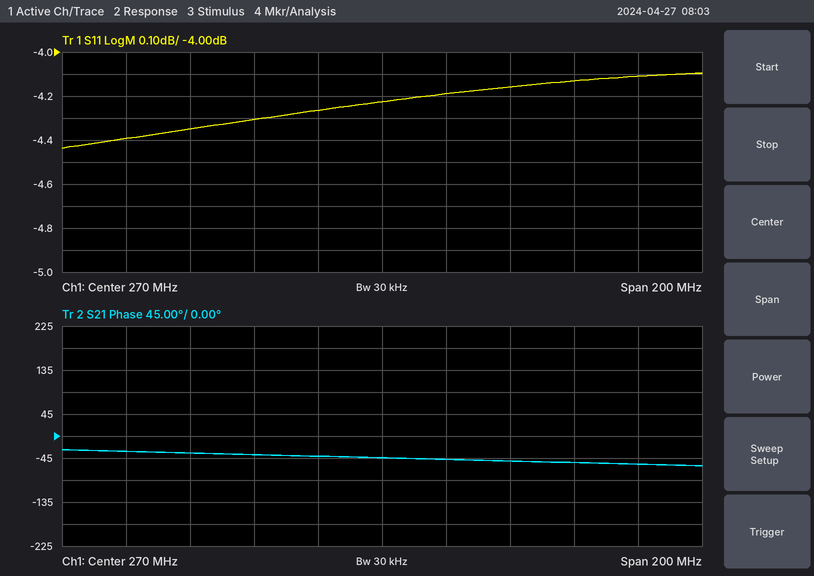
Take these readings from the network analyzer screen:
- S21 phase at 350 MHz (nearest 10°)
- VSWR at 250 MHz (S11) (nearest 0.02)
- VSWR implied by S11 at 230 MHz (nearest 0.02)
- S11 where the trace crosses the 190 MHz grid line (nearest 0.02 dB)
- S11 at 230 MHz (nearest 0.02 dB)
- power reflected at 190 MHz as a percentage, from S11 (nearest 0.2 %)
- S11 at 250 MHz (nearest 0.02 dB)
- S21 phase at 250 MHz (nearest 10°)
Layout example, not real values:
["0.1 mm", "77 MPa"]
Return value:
["-60°", "4.16", "4.12", "-4.40 dB", "-4.30 dB", "36.4 %", "-4.26 dB", "-40°"]
